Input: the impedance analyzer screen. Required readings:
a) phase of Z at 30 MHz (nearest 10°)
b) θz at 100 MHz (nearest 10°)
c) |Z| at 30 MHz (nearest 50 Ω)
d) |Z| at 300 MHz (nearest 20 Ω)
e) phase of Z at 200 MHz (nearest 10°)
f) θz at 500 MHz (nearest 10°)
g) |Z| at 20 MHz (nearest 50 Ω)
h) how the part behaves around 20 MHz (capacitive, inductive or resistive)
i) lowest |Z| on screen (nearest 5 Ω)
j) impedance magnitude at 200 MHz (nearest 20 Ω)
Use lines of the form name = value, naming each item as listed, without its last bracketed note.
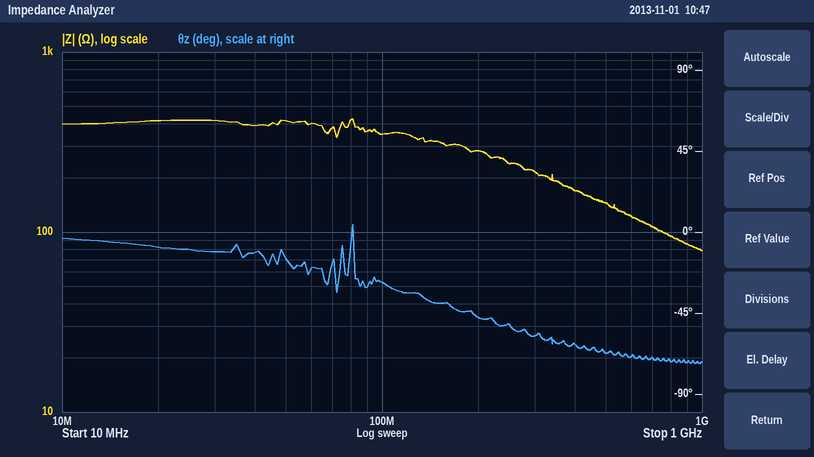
phase of Z at 30 MHz = -10°
θz at 100 MHz = -30°
|Z| at 30 MHz = 400 Ω
|Z| at 300 MHz = 220 Ω
phase of Z at 200 MHz = -50°
θz at 500 MHz = -70°
|Z| at 20 MHz = 400 Ω
how the part behaves around 20 MHz = resistive
lowest |Z| on screen = 80 Ω
impedance magnitude at 200 MHz = 280 Ω
